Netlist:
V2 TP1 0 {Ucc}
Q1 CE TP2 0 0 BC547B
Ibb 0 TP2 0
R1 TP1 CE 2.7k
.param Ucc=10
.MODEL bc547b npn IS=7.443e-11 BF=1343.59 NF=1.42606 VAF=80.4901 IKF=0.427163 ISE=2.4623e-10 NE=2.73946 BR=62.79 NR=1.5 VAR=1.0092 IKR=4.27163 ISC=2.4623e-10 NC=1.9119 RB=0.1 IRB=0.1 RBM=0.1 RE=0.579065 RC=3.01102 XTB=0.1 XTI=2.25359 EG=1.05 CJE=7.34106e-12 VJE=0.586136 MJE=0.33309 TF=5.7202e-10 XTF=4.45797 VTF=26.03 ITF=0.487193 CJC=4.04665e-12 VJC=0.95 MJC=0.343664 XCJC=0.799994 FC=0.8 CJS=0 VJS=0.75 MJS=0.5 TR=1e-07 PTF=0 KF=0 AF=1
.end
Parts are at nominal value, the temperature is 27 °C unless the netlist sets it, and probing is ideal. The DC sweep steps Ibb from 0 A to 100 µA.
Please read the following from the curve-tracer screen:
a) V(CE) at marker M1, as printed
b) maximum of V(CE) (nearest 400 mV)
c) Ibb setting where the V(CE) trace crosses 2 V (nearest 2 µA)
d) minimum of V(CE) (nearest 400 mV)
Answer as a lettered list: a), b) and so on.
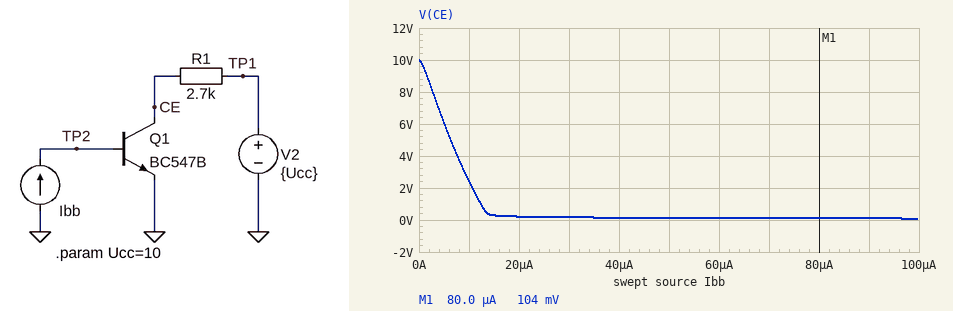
a) 104 mV
b) 10.0 V
c) 10 µA
d) 0 V
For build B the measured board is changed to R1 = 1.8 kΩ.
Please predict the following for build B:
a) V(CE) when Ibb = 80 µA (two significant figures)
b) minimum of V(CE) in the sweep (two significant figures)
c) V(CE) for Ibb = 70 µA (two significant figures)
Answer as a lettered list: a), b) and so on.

a) 130 mV
b) 120 mV
c) 140 mV
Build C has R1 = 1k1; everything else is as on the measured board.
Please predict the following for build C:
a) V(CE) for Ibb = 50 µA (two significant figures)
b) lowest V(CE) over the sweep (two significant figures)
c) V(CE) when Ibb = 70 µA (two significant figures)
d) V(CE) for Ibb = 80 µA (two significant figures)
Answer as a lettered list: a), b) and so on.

a) 230 mV
b) 160 mV
c) 190 mV
d) 180 mV
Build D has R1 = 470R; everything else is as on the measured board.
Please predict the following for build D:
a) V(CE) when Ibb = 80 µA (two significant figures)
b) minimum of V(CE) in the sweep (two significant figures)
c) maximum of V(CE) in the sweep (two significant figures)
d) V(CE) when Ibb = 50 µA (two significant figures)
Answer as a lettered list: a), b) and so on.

a) 1.3 V
b) 410 mV
c) 10 V
d) 3.5 V
